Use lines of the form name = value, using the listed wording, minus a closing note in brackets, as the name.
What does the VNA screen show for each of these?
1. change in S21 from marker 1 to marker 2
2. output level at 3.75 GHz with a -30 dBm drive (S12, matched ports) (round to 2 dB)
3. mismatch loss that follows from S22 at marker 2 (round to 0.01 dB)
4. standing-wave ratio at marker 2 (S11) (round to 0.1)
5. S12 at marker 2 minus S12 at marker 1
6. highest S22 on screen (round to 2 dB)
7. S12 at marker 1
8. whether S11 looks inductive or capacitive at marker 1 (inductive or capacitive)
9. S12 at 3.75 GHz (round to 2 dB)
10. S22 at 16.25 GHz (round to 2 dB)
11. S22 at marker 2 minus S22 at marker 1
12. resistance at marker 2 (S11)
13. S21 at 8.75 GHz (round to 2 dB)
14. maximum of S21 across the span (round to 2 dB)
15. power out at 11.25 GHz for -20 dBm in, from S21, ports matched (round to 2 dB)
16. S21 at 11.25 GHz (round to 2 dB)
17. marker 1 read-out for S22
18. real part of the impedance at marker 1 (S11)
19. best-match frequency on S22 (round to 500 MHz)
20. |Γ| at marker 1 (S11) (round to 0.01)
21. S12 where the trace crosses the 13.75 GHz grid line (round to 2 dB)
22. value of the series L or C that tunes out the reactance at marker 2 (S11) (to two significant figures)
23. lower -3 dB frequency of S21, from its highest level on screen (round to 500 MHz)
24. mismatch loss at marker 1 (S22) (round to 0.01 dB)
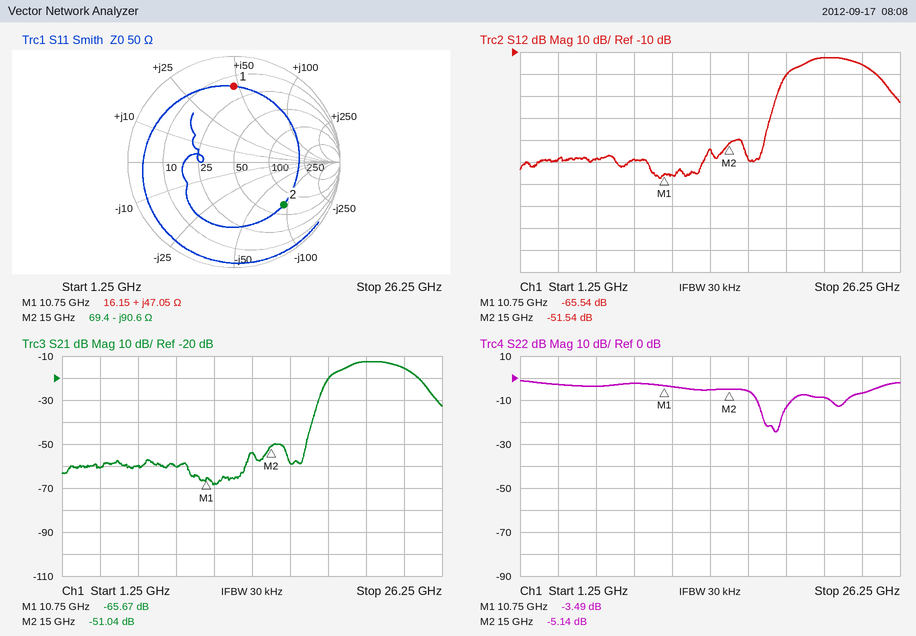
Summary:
change in S21 from marker 1 to marker 2 = 14.63 dB
output level at 3.75 GHz with a -30 dBm drive (S12, matched ports) = -88 dBm
mismatch loss that follows from S22 at marker 2 = 1.59 dB
standing-wave ratio at marker 2 (S11) = 4.2
S12 at marker 2 minus S12 at marker 1 = 14.00 dB
highest S22 on screen = -2 dB
S12 at marker 1 = -65.54 dB
whether S11 looks inductive or capacitive at marker 1 = inductive
S12 at 3.75 GHz = -58 dB
S22 at 16.25 GHz = -6 dB
S22 at marker 2 minus S22 at marker 1 = -1.65 dB
resistance at marker 2 = 69.4 Ω
S21 at 8.75 GHz = -60 dB
maximum of S21 across the span = -12 dB
power out at 11.25 GHz for -20 dBm in, from S21, ports matched = -88 dBm
S21 at 11.25 GHz = -68 dB
marker 1 read-out for S22 = -3.49 dB
real part of the impedance at marker 1 = 16.15 Ω
best-match frequency on S22 = 18.0 GHz
|Γ| at marker 1 (S11) = 0.71
S12 where the trace crosses the 13.75 GHz grid line = -54 dB
value of the series L or C that tunes out the reactance at marker 2 (S11) = 960 pH
lower -3 dB frequency of S21, from its highest level on screen = 20.0 GHz
mismatch loss at marker 1 (S22) = 2.58 dB
